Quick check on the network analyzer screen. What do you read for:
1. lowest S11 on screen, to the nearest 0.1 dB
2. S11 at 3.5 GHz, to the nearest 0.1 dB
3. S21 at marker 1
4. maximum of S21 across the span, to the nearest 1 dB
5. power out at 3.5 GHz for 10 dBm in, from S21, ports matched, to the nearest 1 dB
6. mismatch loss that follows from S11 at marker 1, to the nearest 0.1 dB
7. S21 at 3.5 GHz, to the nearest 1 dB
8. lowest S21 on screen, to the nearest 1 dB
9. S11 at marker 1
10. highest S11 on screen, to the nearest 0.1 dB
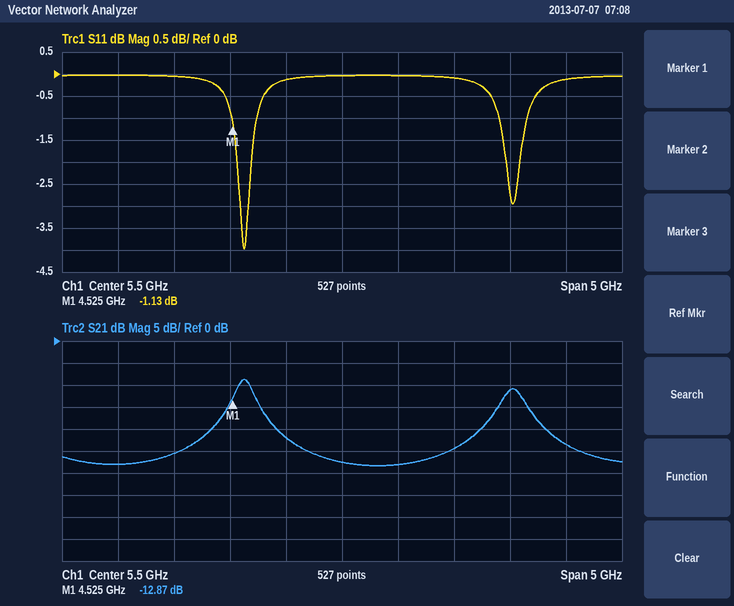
-4.0 dB
0.0 dB
-12.87 dB
-9 dB
-18 dBm
6.4 dB
-28 dB
-28 dB
-1.13 dB
0.0 dB
